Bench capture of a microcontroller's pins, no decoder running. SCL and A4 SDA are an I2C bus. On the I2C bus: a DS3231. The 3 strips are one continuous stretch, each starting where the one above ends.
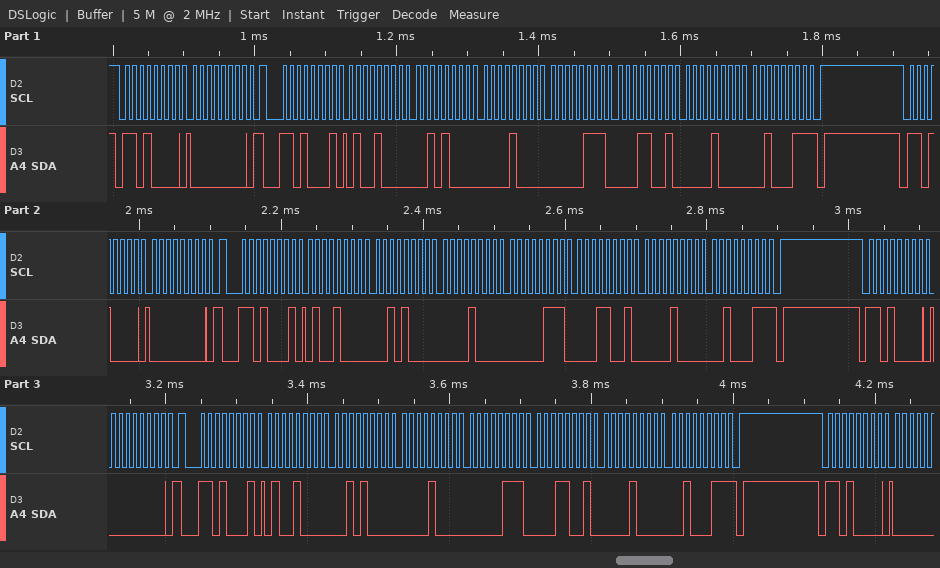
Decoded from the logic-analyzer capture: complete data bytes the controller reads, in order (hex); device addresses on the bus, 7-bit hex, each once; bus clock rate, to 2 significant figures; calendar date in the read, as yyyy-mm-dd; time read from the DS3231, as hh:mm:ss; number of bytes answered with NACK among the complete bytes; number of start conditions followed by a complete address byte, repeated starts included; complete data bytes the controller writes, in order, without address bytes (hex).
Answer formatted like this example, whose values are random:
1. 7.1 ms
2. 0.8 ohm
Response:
1. 48 28 08 07 19 08 23 48 28 08 07 19 08 23 48 28 08 07 19 08 23
2. 0x68
3. 100 kHz
4. 2023-08-19
5. 08:28:48
6. 3
7. 7
8. 00 00 00
